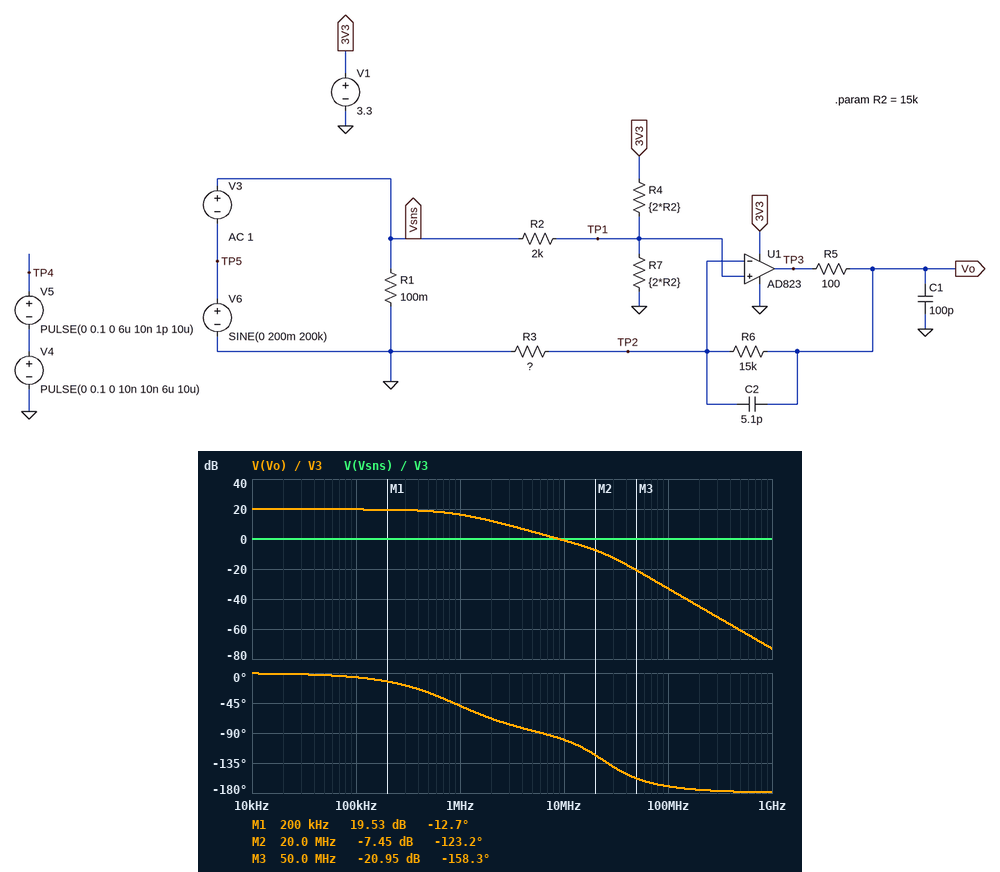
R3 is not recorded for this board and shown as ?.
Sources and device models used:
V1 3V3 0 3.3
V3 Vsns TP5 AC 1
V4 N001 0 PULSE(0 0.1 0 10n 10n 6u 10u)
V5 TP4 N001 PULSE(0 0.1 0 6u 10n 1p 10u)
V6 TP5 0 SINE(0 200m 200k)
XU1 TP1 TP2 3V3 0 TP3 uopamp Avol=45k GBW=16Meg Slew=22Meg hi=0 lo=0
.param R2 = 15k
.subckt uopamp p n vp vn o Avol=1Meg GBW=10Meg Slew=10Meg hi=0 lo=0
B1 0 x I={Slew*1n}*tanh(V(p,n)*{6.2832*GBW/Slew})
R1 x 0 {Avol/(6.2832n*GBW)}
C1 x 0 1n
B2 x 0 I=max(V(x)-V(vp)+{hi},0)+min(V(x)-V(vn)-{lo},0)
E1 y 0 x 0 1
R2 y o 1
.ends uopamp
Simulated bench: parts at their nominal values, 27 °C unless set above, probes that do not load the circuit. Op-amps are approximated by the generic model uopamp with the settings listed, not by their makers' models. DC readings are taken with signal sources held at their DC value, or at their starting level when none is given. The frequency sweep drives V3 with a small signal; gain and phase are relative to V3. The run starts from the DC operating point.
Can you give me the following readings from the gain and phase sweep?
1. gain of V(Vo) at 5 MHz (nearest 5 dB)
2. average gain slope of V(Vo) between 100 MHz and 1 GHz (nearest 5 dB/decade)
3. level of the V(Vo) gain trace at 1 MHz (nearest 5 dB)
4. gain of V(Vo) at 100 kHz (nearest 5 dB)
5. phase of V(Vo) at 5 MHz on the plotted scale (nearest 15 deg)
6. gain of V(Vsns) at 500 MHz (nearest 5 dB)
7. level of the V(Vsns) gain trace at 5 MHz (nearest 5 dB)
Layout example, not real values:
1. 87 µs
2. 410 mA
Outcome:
1. 5 dB
2. -40 dB/decade
3. 15 dB
4. 20 dB
5. -90 deg
6. 0 dB
7. 0 dB
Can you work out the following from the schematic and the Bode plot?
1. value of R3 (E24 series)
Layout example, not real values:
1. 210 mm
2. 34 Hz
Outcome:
1. 1.5 kΩ
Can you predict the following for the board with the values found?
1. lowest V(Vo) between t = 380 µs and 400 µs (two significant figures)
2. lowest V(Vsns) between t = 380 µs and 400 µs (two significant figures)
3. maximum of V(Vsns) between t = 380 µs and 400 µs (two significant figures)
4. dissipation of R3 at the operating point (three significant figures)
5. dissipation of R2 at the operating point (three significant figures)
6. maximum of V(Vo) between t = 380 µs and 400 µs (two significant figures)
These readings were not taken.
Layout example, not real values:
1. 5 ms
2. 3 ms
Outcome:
1. 240 mV
2. -200 mV
3. 200 mV
4. 25.1 µW
5. 18.8 µW
6. 3.3 V
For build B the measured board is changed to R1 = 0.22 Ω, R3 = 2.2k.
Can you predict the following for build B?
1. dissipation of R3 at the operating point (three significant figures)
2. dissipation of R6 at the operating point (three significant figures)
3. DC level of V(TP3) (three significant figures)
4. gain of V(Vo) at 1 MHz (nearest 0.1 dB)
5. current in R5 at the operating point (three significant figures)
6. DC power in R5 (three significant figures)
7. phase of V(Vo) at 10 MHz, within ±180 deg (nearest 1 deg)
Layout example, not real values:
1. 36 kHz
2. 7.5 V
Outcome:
1. 17.1 µW
2. 117 µW
3. 1.53 V
4. 14.2 dB
5. 88.2 µA
6. 778 nW
7. -92 deg
